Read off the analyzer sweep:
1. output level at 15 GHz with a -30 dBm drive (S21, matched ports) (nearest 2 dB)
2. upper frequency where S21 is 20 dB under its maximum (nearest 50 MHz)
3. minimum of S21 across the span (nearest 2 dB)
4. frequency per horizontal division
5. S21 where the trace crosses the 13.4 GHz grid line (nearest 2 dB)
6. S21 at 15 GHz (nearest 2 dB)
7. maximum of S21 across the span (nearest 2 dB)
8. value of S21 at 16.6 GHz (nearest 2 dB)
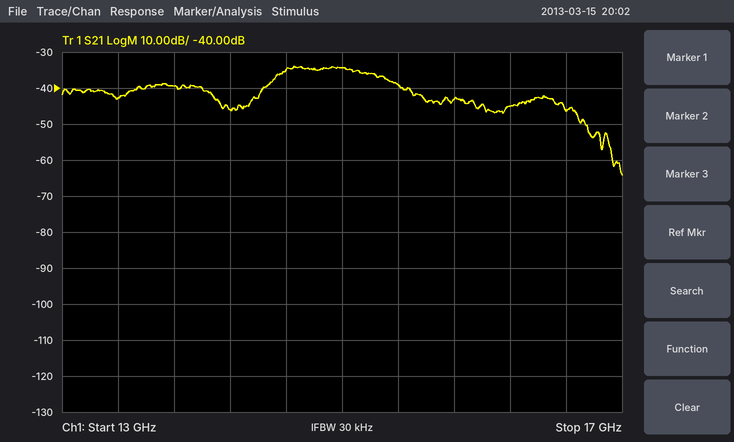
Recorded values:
-64 dBm
16.85 GHz
-64 dB
400 MHz
-42 dB
-34 dB
-34 dB
-46 dB
